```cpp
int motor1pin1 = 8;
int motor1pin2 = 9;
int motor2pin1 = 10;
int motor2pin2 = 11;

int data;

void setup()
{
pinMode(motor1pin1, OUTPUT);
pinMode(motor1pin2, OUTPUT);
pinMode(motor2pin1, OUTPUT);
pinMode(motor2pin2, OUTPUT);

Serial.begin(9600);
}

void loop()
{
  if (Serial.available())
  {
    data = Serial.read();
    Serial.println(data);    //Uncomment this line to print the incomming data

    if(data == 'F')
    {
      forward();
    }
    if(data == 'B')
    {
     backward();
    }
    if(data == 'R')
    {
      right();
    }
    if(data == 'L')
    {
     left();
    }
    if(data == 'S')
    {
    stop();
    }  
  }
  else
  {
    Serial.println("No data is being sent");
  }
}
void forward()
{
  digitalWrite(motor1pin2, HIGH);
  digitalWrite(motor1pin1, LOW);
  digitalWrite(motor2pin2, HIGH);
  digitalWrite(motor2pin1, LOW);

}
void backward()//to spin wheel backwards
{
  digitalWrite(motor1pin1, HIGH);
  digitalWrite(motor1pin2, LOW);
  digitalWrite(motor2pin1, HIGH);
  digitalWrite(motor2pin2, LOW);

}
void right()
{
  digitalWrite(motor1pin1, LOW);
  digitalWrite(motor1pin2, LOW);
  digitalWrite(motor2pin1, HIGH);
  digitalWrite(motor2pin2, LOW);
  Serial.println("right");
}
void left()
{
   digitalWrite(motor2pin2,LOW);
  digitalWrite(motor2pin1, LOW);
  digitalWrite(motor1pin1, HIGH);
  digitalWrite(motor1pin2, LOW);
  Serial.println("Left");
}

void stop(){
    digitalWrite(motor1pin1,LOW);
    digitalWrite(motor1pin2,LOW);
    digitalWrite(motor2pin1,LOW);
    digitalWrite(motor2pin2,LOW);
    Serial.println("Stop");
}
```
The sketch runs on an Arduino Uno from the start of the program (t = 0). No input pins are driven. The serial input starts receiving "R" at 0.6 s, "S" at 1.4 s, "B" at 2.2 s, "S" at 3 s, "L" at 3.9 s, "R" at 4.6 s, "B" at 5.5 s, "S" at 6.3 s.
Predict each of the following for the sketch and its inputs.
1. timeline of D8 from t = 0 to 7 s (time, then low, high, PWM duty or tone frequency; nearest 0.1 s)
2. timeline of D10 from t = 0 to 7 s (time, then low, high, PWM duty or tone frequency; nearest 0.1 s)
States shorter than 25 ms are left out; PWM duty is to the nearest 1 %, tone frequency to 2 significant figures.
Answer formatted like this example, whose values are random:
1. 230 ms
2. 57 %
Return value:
1. 0 s low; 2.2 s high; 3 s low; 3.9 s high; 4.6 s low; 5.5 s high; 6.3 s low
2. 0 s low; 0.6 s high; 1.4 s low; 2.2 s high; 3 s low; 4.6 s high; 6.3 s low
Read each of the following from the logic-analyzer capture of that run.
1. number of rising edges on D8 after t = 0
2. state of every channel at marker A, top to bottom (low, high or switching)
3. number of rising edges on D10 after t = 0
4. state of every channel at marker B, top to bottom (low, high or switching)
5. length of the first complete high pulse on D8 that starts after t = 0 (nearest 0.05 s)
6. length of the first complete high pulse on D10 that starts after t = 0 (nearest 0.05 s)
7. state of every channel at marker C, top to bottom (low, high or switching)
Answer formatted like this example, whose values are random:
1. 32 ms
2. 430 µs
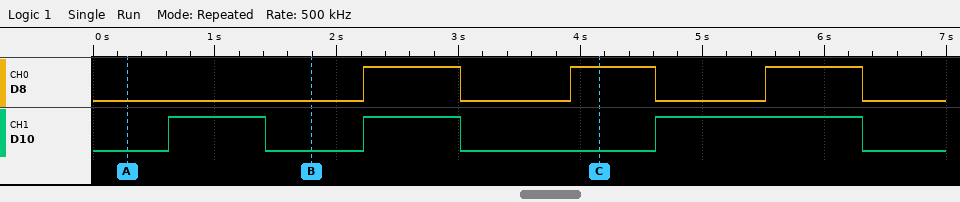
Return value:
1. 3
2. D8 low, D10 low
3. 3
4. D8 low, D10 low
5. 0.80 s
6. 0.80 s
7. D8 high, D10 low
